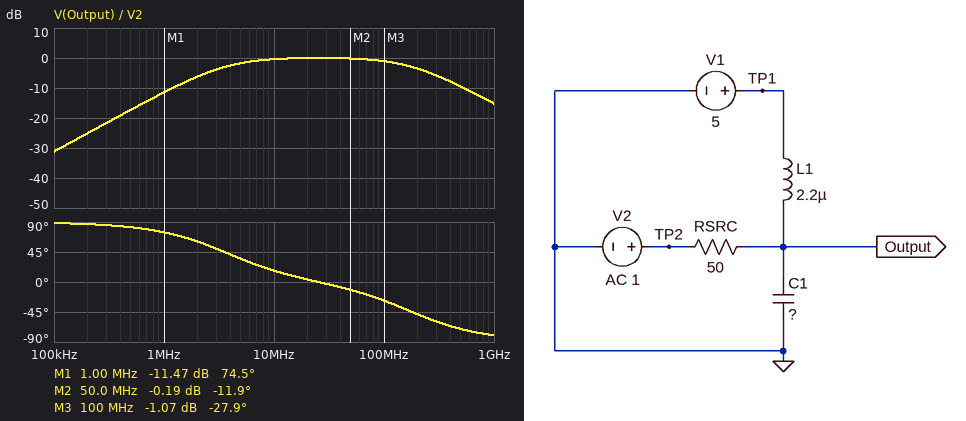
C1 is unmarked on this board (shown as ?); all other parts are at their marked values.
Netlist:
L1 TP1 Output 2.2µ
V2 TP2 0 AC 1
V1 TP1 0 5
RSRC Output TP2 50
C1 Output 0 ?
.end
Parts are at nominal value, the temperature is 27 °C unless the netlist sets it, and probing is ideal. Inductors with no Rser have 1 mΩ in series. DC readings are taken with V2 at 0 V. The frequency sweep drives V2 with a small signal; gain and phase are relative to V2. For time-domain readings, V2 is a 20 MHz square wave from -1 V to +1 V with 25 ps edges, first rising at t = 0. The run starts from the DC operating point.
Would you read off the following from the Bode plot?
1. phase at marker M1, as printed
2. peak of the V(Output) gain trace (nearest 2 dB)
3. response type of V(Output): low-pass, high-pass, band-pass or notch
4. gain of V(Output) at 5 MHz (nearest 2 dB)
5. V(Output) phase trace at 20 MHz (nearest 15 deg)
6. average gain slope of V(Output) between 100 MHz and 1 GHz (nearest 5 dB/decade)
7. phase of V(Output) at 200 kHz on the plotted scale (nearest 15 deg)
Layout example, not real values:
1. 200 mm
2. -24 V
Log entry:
1. 74.5 deg
2. 0 dB
3. band-pass
4. -2 dB
5. 0 deg
6. -15 dB/decade
7. 90 deg
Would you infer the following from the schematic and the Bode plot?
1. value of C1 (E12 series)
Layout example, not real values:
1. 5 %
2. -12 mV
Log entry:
1. 18 pF
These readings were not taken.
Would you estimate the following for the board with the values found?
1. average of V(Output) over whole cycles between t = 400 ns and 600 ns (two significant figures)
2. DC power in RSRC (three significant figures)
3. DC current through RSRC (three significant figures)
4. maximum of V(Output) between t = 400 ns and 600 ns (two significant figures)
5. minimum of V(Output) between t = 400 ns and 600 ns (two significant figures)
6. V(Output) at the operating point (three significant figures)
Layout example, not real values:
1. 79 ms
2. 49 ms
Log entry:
1. 5.0 V
2. 500 mW
3. 100 mA
4. 6.2 V
5. 3.8 V
6. 5.00 V
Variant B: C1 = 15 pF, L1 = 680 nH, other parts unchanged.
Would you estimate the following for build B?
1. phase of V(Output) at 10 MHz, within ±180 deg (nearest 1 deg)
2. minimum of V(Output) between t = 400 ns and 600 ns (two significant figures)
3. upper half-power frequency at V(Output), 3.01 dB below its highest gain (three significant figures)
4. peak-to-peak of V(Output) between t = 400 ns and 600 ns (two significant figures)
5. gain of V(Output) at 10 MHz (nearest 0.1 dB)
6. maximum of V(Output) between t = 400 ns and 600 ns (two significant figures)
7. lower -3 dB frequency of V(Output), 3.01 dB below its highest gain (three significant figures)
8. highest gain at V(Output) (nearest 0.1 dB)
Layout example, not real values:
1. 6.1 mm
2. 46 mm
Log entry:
1. 48 deg
2. 3.5 V
3. 223 MHz
4. 3.1 V
5. -3.5 dB
6. 6.5 V
7. 11.1 MHz
8. 0 dB
